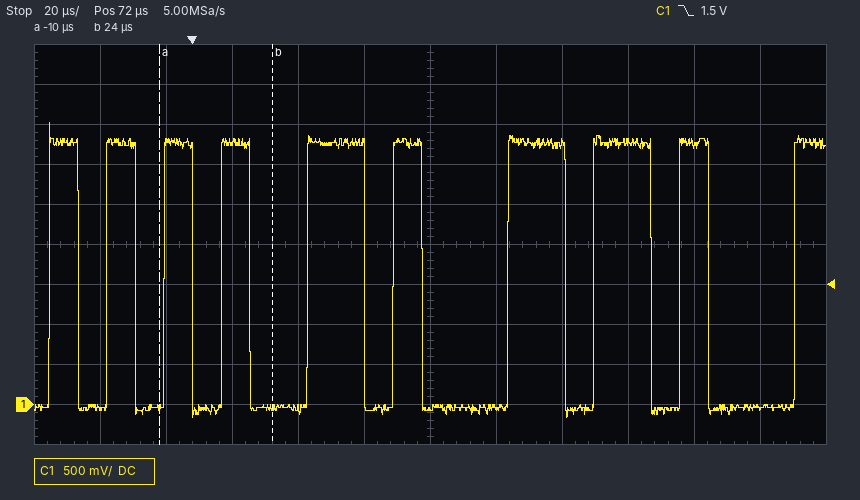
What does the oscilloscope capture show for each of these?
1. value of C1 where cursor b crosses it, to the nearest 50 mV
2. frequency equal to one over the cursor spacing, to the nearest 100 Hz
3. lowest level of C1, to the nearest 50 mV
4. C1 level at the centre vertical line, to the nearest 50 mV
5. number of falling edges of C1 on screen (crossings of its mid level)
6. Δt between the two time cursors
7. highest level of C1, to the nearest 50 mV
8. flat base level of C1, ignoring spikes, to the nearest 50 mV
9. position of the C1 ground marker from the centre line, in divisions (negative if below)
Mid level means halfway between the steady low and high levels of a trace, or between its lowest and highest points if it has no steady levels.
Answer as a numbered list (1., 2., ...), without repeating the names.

1. -50 mV
2. 29.4 kHz
3. -150 mV
4. -50 mV
5. 9
6. 34 µs
7. 3.50 V
8. -50 mV
9. -4.0 div
